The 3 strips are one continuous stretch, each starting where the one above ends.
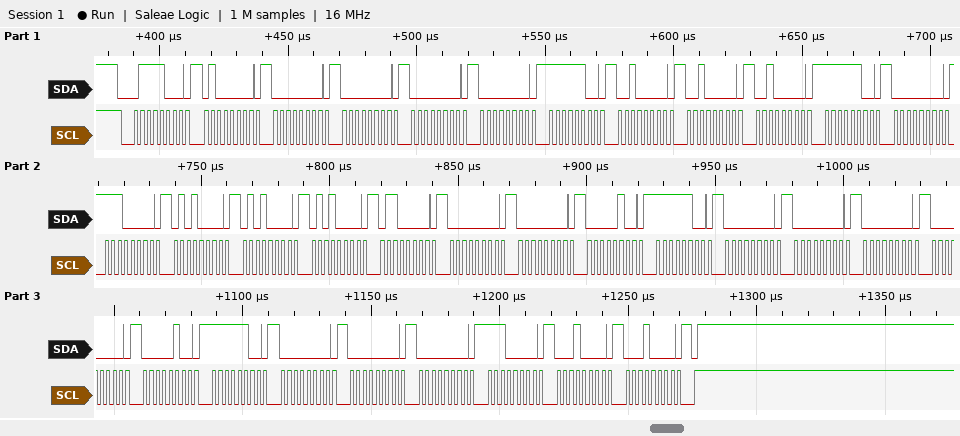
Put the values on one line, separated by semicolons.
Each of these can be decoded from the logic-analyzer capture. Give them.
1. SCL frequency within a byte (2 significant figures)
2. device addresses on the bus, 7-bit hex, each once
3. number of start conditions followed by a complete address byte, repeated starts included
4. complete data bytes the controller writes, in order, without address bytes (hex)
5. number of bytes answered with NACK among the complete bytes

400 kHz; 0x3C; 1; 40 00 00 00 00 FC 20 20 20 FC 00 E0 50 50 50 60 00 00 04 FC 00 00 00 00 04 FC 00 00 00 E0 10 10; 0
